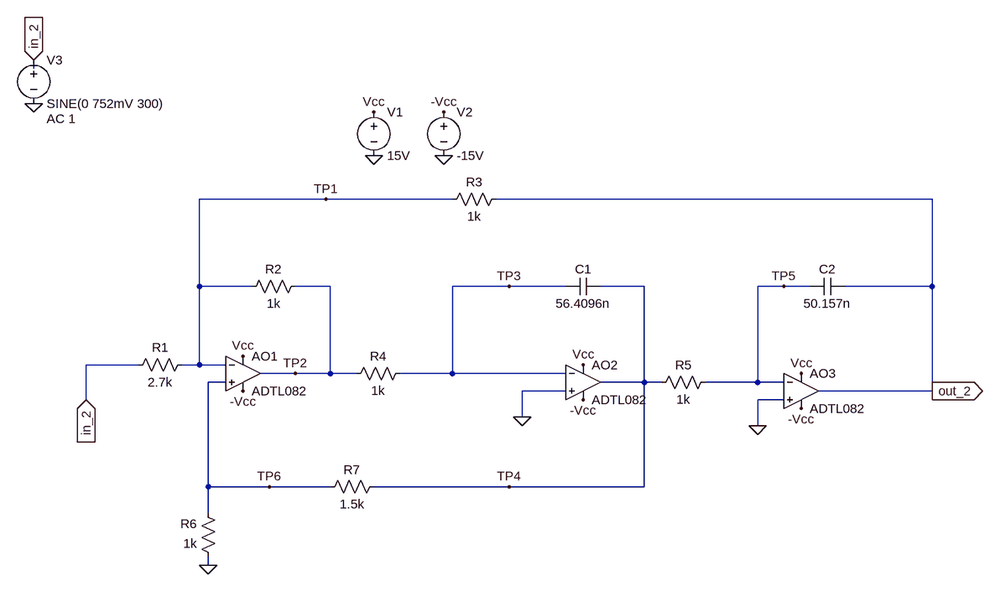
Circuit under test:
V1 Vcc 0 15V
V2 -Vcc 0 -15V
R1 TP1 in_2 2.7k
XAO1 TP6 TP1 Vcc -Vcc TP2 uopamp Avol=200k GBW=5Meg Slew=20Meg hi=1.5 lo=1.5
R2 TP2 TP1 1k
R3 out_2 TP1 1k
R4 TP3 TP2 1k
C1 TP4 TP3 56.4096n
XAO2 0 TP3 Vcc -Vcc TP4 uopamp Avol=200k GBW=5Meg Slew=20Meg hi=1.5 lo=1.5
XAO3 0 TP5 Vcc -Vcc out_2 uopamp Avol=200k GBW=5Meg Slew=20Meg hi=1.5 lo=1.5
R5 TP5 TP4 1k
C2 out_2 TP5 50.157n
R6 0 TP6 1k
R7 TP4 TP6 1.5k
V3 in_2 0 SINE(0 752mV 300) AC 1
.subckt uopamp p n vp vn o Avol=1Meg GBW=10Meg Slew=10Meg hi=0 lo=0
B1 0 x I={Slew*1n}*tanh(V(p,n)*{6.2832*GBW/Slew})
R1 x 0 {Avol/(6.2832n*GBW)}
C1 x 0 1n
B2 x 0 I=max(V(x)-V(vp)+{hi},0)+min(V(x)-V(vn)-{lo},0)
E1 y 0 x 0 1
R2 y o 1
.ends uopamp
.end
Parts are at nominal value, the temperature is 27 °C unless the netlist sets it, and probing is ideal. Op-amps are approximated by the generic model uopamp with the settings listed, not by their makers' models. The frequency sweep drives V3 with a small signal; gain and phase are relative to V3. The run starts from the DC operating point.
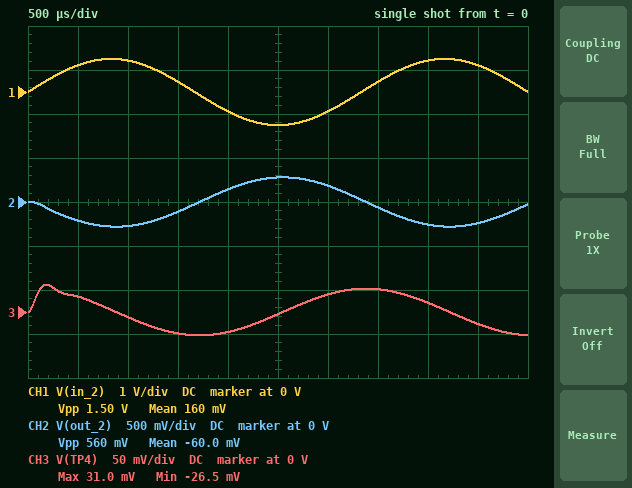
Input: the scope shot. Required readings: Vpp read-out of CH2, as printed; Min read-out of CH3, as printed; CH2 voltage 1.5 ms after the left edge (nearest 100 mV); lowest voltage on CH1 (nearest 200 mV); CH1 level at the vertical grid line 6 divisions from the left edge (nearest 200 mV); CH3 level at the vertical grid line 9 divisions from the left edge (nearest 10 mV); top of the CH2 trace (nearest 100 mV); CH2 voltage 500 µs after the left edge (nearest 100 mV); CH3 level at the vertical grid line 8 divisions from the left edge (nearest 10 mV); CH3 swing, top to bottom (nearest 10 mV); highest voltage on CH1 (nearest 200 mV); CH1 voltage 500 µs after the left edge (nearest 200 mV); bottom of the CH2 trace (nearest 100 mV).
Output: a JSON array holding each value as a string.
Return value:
["560 mV", "-26.5 mV", "-100 mV", "-800 mV", "-400 mV", "-10 mV", "300 mV", "-200 mV", "10 mV", "60 mV", "800 mV", "600 mV", "-300 mV"]
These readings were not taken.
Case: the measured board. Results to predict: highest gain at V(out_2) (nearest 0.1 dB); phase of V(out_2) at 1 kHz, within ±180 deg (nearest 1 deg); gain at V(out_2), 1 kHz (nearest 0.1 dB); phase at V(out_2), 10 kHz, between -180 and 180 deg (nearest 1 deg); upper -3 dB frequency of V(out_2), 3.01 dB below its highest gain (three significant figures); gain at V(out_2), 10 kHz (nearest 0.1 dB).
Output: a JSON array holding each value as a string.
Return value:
["-6.7 dB", "161 deg", "-8.1 dB", "16 deg", "3.54 kHz", "-29.1 dB"]
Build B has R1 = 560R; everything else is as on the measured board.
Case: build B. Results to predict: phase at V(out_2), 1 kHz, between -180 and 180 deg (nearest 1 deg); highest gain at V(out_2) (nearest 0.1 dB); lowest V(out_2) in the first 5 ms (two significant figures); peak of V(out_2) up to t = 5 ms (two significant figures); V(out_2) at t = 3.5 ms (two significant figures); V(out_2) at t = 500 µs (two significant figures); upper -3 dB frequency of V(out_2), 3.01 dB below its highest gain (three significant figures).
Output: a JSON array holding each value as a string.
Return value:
["152 deg", "5.0 dB", "-1.3 V", "1.3 V", "-230 mV", "-960 mV", "2.97 kHz"]
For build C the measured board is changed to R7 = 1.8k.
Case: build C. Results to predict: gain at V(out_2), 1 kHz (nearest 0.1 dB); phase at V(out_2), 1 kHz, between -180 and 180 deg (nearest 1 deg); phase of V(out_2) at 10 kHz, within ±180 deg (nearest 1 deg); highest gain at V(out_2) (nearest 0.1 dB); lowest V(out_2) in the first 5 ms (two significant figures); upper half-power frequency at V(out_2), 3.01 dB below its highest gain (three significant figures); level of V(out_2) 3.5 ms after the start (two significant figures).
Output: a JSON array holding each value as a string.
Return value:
["-8.0 dB", "163 deg", "14 deg", "-5.9 dB", "-280 mV", "3.56 kHz", "-65 mV"]
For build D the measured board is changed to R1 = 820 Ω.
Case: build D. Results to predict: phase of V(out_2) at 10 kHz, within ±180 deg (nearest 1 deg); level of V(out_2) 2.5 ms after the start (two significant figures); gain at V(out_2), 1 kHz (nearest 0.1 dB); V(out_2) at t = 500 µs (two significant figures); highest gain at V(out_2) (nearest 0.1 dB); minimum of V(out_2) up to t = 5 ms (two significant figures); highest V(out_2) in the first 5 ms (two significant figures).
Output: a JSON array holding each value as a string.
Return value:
["21 deg", "910 mV", "1.9 dB", "-670 mV", "2.0 dB", "-920 mV", "920 mV"]
